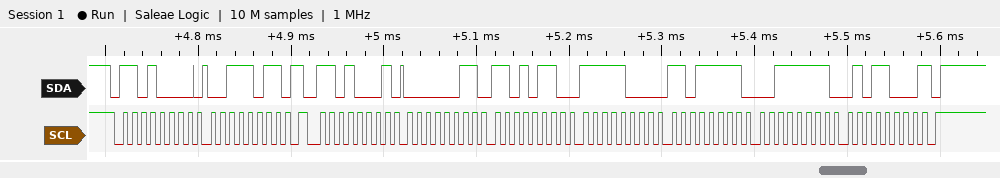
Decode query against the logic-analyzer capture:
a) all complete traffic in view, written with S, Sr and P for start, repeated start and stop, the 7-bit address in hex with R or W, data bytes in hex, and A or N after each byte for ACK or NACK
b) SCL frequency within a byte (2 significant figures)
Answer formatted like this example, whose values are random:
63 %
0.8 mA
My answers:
S 68W A 3B A Sr 68R A 03 A D6 A F8 A DF A 3F A 58 N P
100 kHz
